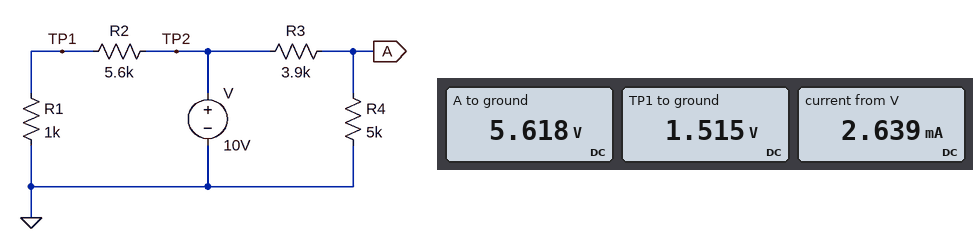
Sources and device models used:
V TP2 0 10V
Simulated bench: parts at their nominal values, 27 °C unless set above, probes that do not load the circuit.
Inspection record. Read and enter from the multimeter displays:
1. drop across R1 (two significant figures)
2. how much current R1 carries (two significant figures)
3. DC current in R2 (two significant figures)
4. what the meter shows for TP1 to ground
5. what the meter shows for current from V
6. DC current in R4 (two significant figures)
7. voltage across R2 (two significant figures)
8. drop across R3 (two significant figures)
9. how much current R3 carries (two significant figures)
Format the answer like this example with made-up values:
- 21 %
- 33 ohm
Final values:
- 1.5 V
- 1.5 mA
- 1.5 mA
- 1.515 V
- 2.639 mA
- 1.1 mA
- 8.5 V
- 4.4 V
- 1.1 mA
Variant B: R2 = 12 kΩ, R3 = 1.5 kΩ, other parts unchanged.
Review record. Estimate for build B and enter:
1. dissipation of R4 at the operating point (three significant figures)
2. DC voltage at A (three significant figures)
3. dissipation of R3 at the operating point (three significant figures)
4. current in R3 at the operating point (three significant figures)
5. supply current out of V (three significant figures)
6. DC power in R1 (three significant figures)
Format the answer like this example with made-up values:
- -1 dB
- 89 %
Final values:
- 11.8 mW
- 7.69 V
- 3.55 mW
- 1.54 mA
- 2.31 mA
- 592 µW
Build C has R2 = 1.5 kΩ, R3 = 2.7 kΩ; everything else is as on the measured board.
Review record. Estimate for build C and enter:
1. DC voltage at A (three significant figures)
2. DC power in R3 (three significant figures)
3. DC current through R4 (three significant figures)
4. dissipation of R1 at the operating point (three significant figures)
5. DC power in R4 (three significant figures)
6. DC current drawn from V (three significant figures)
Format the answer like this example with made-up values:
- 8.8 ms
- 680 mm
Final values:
- 6.49 V
- 4.55 mW
- 1.30 mA
- 16.0 mW
- 8.43 mW
- 5.30 mA
